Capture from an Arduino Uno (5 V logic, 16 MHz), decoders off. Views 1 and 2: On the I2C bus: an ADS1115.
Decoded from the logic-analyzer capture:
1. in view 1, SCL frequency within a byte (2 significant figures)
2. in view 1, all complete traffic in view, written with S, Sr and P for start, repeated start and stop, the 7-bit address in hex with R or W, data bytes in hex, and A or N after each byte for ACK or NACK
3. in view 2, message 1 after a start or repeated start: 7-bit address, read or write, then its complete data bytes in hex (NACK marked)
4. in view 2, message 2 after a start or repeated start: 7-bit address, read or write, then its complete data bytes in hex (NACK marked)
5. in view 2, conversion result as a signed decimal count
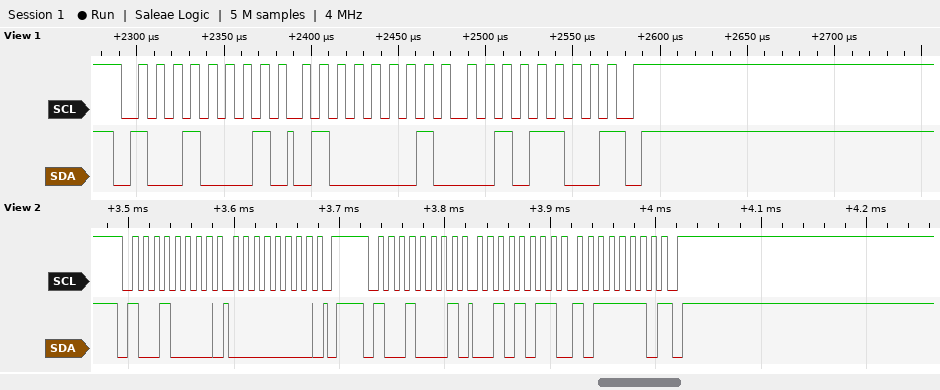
100 kHz
S 48R A 41 A 2C N P
0x48 write: 00
0x48 read: 2B BE NACK
11198
